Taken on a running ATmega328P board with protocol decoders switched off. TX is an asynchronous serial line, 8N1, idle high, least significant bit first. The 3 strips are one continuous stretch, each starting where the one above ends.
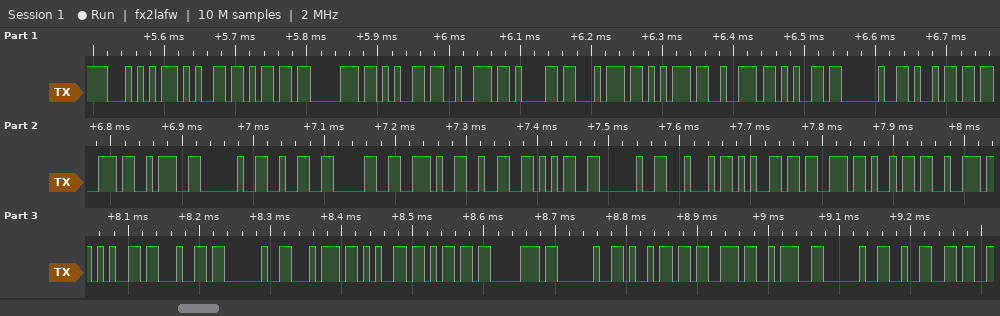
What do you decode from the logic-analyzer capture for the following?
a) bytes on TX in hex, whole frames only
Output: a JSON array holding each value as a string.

["54 65 6D 70 65 72 61 74 75 72 65 20 69 73 3A 20 32 30 2E 32 35 20 44 65 73 69 72 65 64 20 74 65 6D 70 20 69 73 3A 20 32"]
